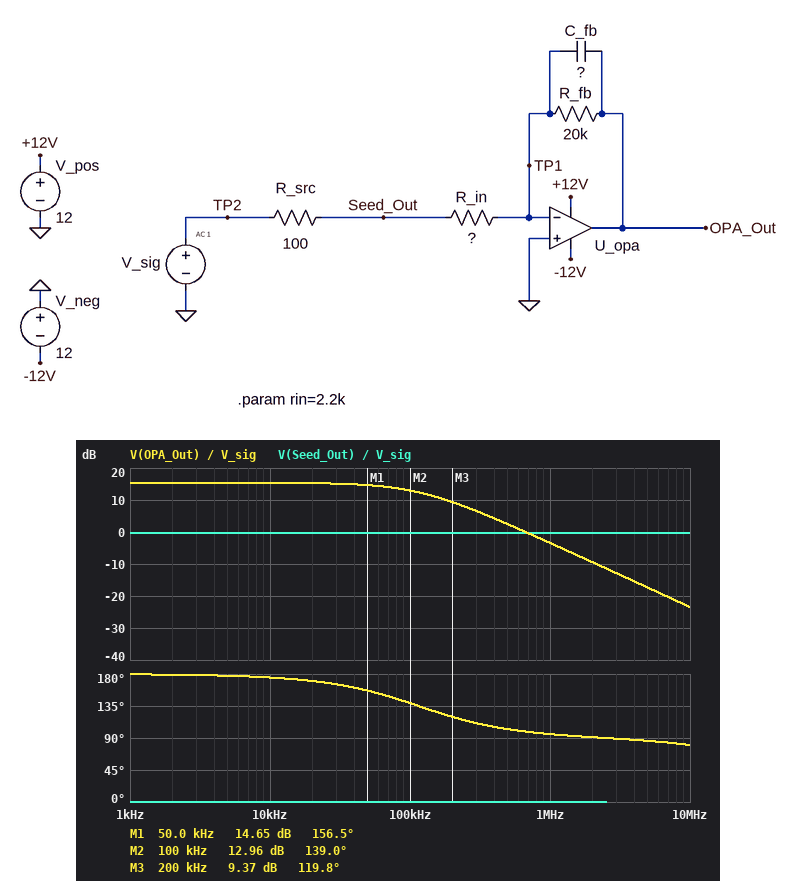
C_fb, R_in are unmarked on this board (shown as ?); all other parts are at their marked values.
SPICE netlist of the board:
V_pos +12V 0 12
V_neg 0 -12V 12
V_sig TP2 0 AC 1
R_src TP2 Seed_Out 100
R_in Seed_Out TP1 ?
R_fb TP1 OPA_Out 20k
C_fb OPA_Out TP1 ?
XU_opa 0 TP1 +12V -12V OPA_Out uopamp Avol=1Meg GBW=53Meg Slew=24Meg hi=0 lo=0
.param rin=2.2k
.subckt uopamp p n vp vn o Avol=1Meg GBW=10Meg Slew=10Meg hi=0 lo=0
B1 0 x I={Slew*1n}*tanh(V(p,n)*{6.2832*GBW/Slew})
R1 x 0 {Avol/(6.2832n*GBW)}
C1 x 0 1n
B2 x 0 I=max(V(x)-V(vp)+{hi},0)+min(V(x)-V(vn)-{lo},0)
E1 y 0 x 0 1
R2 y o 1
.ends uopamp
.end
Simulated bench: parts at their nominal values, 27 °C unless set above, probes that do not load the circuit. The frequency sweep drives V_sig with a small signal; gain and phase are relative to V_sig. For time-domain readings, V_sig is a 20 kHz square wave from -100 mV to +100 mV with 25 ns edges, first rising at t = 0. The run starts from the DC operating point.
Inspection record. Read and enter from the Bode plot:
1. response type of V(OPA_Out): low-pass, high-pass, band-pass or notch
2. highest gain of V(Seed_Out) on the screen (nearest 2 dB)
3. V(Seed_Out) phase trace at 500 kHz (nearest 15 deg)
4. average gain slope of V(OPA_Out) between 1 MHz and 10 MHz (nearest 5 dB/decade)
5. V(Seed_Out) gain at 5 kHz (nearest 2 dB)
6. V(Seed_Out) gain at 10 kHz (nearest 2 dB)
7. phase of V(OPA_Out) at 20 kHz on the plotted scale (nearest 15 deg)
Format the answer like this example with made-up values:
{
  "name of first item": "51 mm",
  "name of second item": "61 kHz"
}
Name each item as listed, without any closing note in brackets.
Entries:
{
  "response type of V(OPA_Out): low-pass, high-pass, band-pass or notch": "low-pass",
  "highest gain of V(Seed_Out) on the screen": "0 dB",
  "V(Seed_Out) phase trace at 500 kHz": "0 deg",
  "average gain slope of V(OPA_Out) between 1 MHz and 10 MHz": "-20 dB/decade",
  "V(Seed_Out) gain at 5 kHz": "0 dB",
  "V(Seed_Out) gain at 10 kHz": "0 dB",
  "phase of V(OPA_Out) at 20 kHz on the plotted scale": "165 deg"
}
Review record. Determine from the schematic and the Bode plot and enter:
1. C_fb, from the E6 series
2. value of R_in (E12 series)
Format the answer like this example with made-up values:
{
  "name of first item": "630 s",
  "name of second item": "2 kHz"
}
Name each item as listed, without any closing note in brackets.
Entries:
{
  "C_fb, from the E6 series": "68 pF",
  "value of R_in": "3.3 kΩ"
}
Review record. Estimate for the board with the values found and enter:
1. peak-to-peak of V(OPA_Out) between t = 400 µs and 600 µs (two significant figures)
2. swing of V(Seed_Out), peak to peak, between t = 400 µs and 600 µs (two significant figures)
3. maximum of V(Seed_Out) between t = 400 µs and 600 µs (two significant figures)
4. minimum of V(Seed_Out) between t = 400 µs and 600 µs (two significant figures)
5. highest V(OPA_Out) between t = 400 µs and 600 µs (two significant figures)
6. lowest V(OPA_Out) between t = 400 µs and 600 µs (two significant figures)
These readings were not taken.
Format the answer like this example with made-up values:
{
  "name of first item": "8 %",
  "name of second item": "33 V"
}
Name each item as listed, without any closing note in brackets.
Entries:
{
  "peak-to-peak of V(OPA_Out) between t = 400 µs and 600 µs": "1.2 V",
  "swing of V(Seed_Out), peak to peak, between t = 400 µs and 600 µs": "190 mV",
  "maximum of V(Seed_Out) between t = 400 µs and 600 µs": "97 mV",
  "minimum of V(Seed_Out) between t = 400 µs and 600 µs": "-97 mV",
  "highest V(OPA_Out) between t = 400 µs and 600 µs": "590 mV",
  "lowest V(OPA_Out) between t = 400 µs and 600 µs": "-590 mV"
}
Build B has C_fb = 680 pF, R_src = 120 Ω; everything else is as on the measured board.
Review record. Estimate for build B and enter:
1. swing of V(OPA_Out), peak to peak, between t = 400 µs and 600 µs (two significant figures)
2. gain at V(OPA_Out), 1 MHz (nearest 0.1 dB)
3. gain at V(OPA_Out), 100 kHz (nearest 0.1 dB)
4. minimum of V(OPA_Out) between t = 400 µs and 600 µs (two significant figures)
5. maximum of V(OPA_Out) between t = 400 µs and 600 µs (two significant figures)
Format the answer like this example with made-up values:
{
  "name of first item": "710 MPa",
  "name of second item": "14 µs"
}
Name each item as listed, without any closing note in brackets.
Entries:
{
  "swing of V(OPA_Out), peak to peak, between t = 400 µs and 600 µs": "850 mV",
  "gain at V(OPA_Out), 1 MHz": "-23.3 dB",
  "gain at V(OPA_Out), 100 kHz": "-3.4 dB",
  "minimum of V(OPA_Out) between t = 400 µs and 600 µs": "-420 mV",
  "maximum of V(OPA_Out) between t = 400 µs and 600 µs": "420 mV"
}
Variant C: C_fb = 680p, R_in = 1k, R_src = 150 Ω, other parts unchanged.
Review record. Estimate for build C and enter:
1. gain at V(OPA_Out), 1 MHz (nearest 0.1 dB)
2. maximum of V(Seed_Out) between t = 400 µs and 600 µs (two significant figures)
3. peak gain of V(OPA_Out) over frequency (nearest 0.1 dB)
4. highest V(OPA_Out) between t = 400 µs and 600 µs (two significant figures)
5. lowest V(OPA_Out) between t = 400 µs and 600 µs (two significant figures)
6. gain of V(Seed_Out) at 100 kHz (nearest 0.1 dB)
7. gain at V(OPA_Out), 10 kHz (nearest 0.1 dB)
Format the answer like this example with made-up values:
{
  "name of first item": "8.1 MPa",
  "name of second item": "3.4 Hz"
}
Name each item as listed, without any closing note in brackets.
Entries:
{
  "gain at V(OPA_Out), 1 MHz": "-13.9 dB",
  "maximum of V(Seed_Out) between t = 400 µs and 600 µs": "87 mV",
  "peak gain of V(OPA_Out) over frequency": "24.8 dB",
  "highest V(OPA_Out) between t = 400 µs and 600 µs": "1.3 V",
  "lowest V(OPA_Out) between t = 400 µs and 600 µs": "-1.3 V",
  "gain of V(Seed_Out) at 100 kHz": "-1.2 dB",
  "gain at V(OPA_Out), 10 kHz": "22.4 dB"
}
